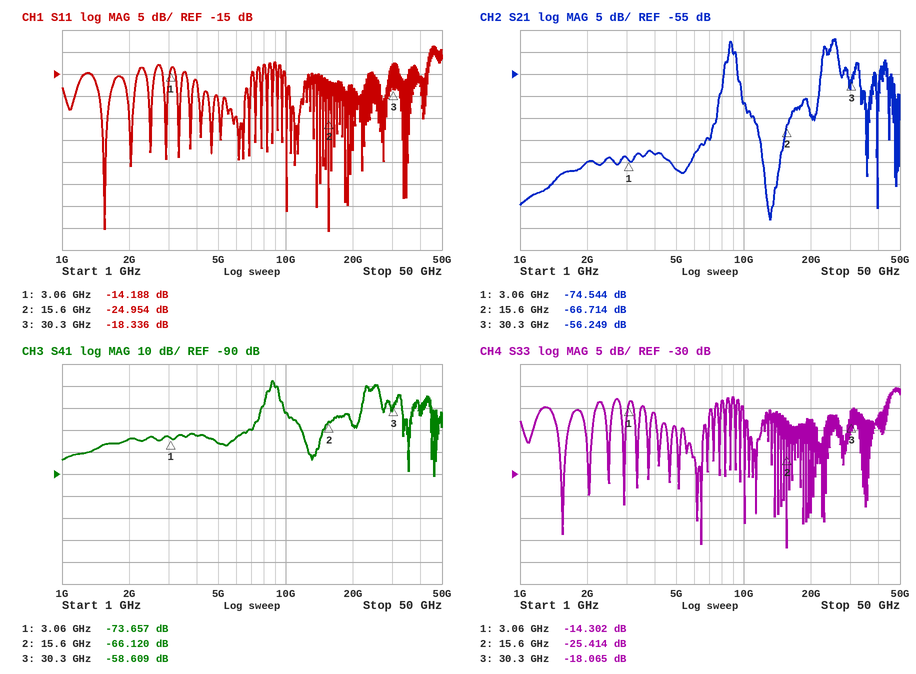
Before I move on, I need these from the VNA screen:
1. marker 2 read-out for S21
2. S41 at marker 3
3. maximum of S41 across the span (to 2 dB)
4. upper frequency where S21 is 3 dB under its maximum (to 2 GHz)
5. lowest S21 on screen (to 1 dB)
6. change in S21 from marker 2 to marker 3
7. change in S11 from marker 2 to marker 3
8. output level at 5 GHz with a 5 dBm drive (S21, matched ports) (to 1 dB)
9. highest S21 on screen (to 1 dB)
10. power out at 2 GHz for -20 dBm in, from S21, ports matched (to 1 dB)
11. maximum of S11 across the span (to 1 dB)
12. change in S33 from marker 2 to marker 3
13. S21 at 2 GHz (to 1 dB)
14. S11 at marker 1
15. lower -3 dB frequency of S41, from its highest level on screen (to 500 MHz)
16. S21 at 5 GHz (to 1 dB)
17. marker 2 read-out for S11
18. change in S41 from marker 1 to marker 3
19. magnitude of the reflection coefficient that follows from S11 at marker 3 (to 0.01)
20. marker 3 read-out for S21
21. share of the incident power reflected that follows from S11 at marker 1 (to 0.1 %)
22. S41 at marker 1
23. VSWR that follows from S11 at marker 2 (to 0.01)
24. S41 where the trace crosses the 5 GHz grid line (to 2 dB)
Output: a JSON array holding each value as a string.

["-66.714 dB", "-58.609 dB", "-48 dB", "26 GHz", "-88 dB", "10.465 dB", "6.618 dB", "-72 dBm", "-47 dB", "-95 dBm", "-9 dB", "7.349 dB", "-75 dB", "-14.188 dB", "8.5 GHz", "-77 dB", "-24.954 dB", "15.048 dB", "0.12", "-56.249 dB", "3.8 %", "-73.657 dB", "1.12", "-76 dB"]
